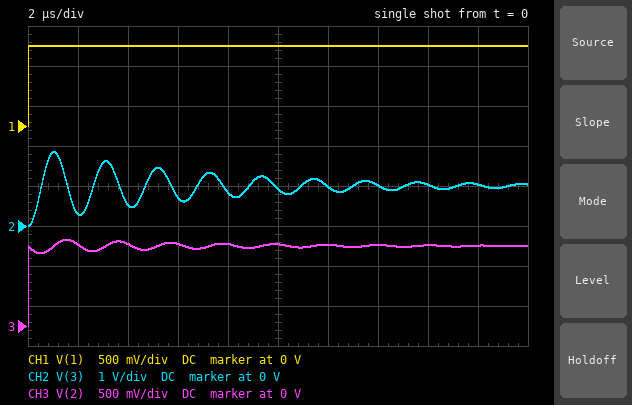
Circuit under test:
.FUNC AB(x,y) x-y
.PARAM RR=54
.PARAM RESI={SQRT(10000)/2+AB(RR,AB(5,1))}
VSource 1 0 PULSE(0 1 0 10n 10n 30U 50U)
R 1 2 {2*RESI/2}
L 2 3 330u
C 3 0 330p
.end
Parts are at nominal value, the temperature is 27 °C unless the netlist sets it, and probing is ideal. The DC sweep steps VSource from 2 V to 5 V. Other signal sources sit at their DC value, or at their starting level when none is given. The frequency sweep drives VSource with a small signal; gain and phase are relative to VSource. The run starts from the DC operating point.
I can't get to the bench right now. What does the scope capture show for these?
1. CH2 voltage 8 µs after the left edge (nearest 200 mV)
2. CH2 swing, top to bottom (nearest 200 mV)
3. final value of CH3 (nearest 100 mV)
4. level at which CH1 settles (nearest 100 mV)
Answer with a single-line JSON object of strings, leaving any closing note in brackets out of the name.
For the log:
{"CH2 voltage 8 µs after the left edge": "800 mV", "CH2 swing, top to bottom": "1.8 V", "final value of CH3": "1.0 V", "level at which CH1 settles": "1.0 V"}
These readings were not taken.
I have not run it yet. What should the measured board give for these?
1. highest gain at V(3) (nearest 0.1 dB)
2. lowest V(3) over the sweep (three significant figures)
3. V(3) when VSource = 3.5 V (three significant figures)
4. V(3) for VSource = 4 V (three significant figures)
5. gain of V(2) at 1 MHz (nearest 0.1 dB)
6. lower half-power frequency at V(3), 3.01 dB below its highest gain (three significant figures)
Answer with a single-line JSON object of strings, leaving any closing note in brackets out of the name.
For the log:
{"highest gain at V(3)": "20.0 dB", "lowest V(3) over the sweep": "2.00 V", "V(3) when VSource = 3.5 V": "3.50 V", "V(3) for VSource = 4 V": "4.00 V", "gain of V(2) at 1 MHz": "0 dB", "lower half-power frequency at V(3), 3.01 dB below its highest gain": "456 kHz"}
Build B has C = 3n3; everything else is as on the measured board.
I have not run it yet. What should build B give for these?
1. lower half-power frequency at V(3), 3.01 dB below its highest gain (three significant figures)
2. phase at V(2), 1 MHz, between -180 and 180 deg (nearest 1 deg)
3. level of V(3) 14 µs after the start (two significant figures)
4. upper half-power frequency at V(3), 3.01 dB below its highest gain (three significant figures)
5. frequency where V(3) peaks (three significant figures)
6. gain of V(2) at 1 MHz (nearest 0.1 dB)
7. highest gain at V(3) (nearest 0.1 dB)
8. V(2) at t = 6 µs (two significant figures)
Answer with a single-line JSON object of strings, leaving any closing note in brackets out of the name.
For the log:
{"lower half-power frequency at V(3), 3.01 dB below its highest gain": "122 kHz", "phase at V(2), 1 MHz, between -180 and 180 deg": "3 deg", "level of V(3) 14 µs after the start": "890 mV", "upper half-power frequency at V(3), 3.01 dB below its highest gain": "171 kHz", "frequency where V(3) peaks": "149 kHz", "gain of V(2) at 1 MHz": "0 dB", "highest gain at V(3)": "10.1 dB", "V(2) at t = 6 µs": "1.1 V"}
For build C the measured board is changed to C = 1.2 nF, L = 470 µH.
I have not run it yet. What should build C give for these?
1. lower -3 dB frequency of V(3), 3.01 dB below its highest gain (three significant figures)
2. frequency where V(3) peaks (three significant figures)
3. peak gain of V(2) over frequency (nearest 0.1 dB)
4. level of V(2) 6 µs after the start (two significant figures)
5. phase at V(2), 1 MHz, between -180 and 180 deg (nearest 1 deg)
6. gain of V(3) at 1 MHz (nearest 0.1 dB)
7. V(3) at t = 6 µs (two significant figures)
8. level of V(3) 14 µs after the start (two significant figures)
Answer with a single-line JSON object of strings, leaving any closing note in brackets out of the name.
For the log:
{"lower -3 dB frequency of V(3), 3.01 dB below its highest gain": "193 kHz", "frequency where V(3) peaks": "211 kHz", "peak gain of V(2) over frequency": "0 dB", "level of V(2) 6 µs after the start": "920 mV", "phase at V(2), 1 MHz, between -180 and 180 deg": "2 deg", "gain of V(3) at 1 MHz": "-26.6 dB", "V(3) at t = 6 µs": "1.0 V", "level of V(3) 14 µs after the start": "790 mV"}
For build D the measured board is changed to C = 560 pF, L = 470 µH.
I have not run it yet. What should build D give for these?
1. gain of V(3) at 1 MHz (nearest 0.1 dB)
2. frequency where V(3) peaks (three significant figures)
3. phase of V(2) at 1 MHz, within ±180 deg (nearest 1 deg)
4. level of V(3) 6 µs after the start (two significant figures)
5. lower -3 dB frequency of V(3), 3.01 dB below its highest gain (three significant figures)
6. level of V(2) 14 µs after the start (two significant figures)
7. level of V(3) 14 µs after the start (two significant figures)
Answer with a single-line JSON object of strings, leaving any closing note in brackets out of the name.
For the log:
{"gain of V(3) at 1 MHz": "-19.5 dB", "frequency where V(3) peaks": "309 kHz", "phase of V(2) at 1 MHz, within ±180 deg": "2 deg", "level of V(3) 6 µs after the start": "690 mV", "lower -3 dB frequency of V(3), 3.01 dB below its highest gain": "292 kHz", "level of V(2) 14 µs after the start": "980 mV", "level of V(3) 14 µs after the start": "1.1 V"}
